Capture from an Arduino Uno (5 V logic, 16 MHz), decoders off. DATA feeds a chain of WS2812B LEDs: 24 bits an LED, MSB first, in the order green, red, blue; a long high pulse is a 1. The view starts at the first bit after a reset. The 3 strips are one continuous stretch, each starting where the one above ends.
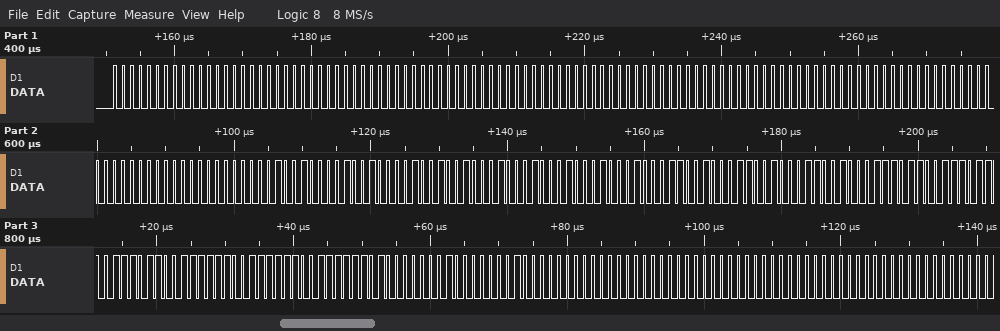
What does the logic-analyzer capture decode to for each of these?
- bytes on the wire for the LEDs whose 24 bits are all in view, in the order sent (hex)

00 00 00 00 00 00 00 00 00 00 00 00 00 00 00 09 09 09 22 22 22 32 32 32 3B 3B 3B 3F 3F 3F 40 40 40 00 00 00 00 00 00
